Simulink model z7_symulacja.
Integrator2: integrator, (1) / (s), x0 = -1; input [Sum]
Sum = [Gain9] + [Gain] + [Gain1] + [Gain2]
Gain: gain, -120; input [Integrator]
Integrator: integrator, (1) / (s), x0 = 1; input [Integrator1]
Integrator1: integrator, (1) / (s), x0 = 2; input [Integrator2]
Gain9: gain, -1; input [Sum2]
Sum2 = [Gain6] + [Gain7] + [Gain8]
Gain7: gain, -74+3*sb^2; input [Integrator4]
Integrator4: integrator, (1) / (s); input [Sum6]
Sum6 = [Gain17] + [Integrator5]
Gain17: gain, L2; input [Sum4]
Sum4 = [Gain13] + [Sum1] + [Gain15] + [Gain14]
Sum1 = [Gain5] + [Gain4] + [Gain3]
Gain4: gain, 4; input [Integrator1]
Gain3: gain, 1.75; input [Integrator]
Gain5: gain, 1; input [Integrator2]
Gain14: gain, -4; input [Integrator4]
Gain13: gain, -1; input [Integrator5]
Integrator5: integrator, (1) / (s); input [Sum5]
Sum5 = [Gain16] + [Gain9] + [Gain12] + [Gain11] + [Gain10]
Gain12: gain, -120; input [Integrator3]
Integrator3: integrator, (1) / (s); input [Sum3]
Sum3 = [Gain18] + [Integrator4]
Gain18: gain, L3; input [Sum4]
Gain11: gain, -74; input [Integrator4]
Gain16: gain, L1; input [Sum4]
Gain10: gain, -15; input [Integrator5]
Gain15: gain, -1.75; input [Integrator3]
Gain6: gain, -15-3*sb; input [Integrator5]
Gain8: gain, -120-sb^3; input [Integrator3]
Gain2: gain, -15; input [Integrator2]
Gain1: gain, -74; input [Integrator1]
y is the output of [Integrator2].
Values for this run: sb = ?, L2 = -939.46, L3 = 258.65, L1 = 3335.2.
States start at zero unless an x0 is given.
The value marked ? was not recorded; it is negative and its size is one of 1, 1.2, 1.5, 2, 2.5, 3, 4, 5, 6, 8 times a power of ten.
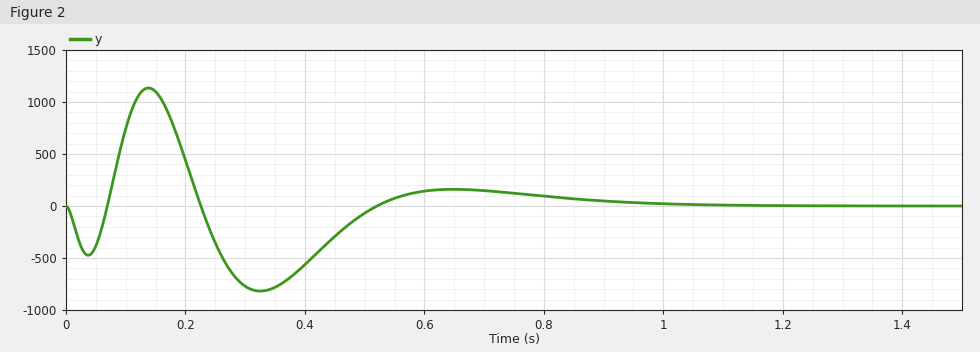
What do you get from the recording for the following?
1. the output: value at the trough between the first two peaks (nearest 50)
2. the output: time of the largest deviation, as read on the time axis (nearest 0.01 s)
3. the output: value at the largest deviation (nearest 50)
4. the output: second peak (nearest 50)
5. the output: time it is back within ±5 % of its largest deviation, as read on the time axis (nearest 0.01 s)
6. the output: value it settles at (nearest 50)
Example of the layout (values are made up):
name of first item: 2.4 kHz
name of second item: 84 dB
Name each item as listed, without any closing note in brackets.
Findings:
the output: value at the trough between the first two peaks: -800
the output: time of the largest deviation, as read on the time axis: 0.14 s
the output: value at the largest deviation: 1150
the output: second peak: 150
the output: time it is back within ±5 % of its largest deviation, as read on the time axis: 0.88 s
the output: value it settles at: 0
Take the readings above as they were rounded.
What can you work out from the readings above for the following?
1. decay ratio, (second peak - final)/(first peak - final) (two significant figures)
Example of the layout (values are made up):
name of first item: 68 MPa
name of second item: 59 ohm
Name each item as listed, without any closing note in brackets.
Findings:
decay ratio, (second peak - final)/(first peak - final): 0.13
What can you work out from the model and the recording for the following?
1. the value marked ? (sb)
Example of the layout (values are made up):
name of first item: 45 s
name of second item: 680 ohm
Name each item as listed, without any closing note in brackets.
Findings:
the value marked ?: -15
